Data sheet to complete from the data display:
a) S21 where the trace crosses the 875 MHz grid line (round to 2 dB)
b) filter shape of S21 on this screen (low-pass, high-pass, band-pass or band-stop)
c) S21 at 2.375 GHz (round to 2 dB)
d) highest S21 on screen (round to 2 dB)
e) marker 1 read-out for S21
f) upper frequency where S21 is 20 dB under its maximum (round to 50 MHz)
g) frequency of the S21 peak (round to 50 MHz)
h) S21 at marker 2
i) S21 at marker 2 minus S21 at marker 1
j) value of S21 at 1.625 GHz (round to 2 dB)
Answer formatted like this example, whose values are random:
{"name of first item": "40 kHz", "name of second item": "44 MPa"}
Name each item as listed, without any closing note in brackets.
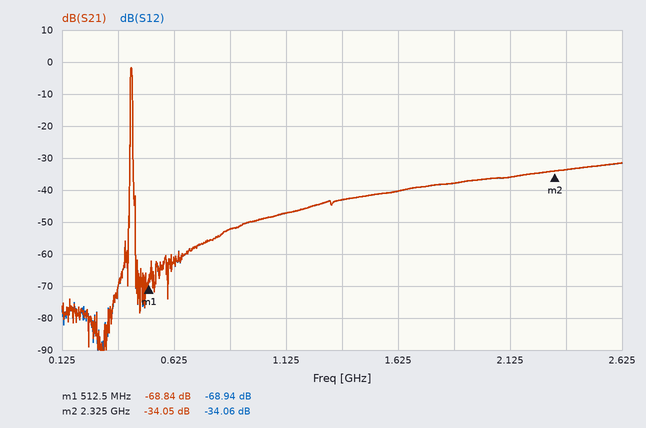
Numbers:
{"S21 where the trace crosses the 875 MHz grid line": "-52 dB", "filter shape of S21 on this screen": "band-pass", "S21 at 2.375 GHz": "-34 dB", "highest S21 on screen": "-2 dB", "marker 1 read-out for S21": "-68.84 dB", "upper frequency where S21 is 20 dB under its maximum": "450 MHz", "frequency of the S21 peak": "450 MHz", "S21 at marker 2": "-34.05 dB", "S21 at marker 2 minus S21 at marker 1": "34.79 dB", "value of S21 at 1.625 GHz": "-40 dB"}
